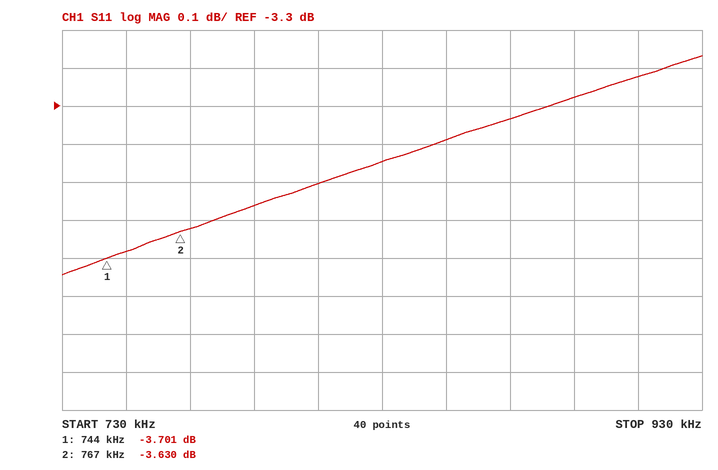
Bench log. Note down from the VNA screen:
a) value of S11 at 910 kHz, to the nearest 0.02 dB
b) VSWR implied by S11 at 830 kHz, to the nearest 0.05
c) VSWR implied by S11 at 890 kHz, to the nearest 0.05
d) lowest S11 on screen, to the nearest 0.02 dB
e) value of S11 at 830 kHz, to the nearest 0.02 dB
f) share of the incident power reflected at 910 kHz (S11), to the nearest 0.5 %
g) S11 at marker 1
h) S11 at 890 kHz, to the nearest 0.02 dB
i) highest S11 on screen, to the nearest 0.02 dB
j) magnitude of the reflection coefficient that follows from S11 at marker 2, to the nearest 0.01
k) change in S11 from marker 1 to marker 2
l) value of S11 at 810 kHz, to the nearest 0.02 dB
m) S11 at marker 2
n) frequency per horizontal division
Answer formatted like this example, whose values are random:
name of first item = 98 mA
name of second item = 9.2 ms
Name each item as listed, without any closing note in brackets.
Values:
value of S11 at 910 kHz, to the nearest 0.02 dB = -3.22 dB
VSWR implied by S11 at 830 kHz, to the nearest 0.05 = 5.10
VSWR implied by S11 at 890 kHz, to the nearest 0.05 = 5.35
lowest S11 on screen, to the nearest 0.02 dB = -3.74 dB
value of S11 at 830 kHz, to the nearest 0.02 dB = -3.44 dB
share of the incident power reflected at 910 kHz (S11), to the nearest 0.5 % = 47.5 %
S11 at marker 1 = -3.701 dB
S11 at 890 kHz, to the nearest 0.02 dB = -3.28 dB
highest S11 on screen, to the nearest 0.02 dB = -3.16 dB
magnitude of the reflection coefficient that follows from S11 at marker 2, to the nearest 0.01 = 0.66
change in S11 from marker 1 to marker 2 = 0.071 dB
value of S11 at 810 kHz, to the nearest 0.02 dB = -3.50 dB
S11 at marker 2 = -3.630 dB
frequency per horizontal division = 20 kHz
